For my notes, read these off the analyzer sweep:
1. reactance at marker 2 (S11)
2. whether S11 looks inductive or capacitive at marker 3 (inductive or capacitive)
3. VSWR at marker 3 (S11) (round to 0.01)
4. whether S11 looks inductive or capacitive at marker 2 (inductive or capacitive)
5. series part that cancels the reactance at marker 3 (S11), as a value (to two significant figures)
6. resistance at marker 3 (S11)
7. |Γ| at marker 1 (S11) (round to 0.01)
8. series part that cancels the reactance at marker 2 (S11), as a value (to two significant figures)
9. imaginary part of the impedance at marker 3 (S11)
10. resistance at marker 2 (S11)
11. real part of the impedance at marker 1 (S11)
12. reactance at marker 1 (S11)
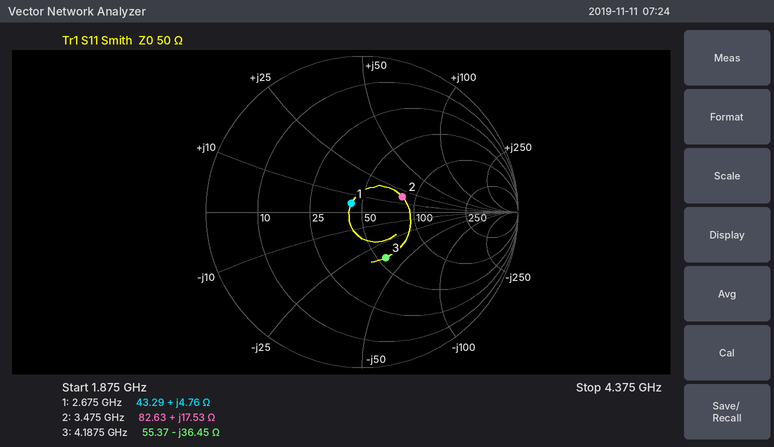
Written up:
+17.53 Ω
capacitive
1.99
inductive
1.4 nH
55.37 Ω
0.09
2.6 pF
-36.45 Ω
82.63 Ω
43.29 Ω
+4.76 Ω
